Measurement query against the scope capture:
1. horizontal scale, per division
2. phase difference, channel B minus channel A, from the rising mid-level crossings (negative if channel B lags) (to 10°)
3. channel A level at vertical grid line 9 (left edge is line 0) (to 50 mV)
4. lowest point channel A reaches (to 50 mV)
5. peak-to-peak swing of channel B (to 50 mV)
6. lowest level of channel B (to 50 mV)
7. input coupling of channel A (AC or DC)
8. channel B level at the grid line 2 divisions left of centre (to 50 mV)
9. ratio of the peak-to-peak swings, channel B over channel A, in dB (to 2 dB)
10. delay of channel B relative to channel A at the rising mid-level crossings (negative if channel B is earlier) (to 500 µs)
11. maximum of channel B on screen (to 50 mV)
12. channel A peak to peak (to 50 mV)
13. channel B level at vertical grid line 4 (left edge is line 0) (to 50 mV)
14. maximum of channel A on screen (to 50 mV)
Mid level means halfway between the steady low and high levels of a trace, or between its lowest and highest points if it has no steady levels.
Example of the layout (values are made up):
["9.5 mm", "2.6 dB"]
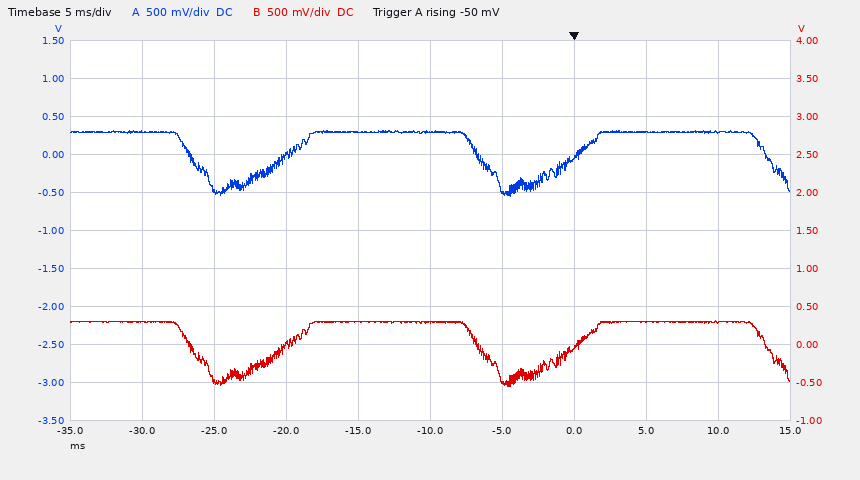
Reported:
["5 ms", "0°", "300 mV", "-550 mV", "850 mV", "-550 mV", "DC", "0 mV", "0 dB", "0.0 ms", "300 mV", "850 mV", "300 mV", "300 mV"]
